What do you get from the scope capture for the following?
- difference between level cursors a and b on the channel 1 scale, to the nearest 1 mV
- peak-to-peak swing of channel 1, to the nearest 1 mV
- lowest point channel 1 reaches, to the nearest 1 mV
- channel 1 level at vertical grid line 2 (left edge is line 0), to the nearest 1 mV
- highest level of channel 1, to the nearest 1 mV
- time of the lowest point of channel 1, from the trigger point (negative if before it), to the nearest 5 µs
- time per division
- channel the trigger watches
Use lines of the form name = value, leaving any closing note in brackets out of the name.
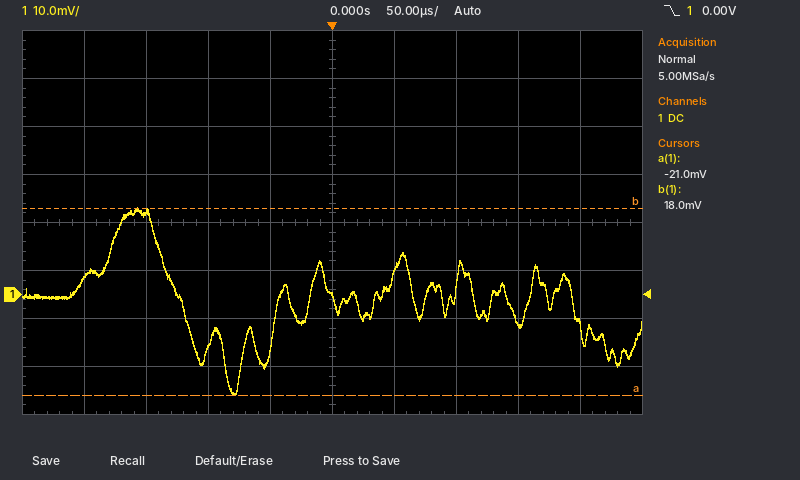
difference between level cursors a and b on the channel 1 scale, to the nearest 1 mV = 39 mV
peak-to-peak swing of channel 1, to the nearest 1 mV = 39 mV
lowest point channel 1 reaches, to the nearest 1 mV = -21 mV
channel 1 level at vertical grid line 2 (left edge is line 0), to the nearest 1 mV = 17 mV
highest level of channel 1, to the nearest 1 mV = 18 mV
time of the lowest point of channel 1, from the trigger point (negative if before it), to the nearest 5 µs = -80 µs
time per division = 50 µs
channel the trigger watches = channel 1
